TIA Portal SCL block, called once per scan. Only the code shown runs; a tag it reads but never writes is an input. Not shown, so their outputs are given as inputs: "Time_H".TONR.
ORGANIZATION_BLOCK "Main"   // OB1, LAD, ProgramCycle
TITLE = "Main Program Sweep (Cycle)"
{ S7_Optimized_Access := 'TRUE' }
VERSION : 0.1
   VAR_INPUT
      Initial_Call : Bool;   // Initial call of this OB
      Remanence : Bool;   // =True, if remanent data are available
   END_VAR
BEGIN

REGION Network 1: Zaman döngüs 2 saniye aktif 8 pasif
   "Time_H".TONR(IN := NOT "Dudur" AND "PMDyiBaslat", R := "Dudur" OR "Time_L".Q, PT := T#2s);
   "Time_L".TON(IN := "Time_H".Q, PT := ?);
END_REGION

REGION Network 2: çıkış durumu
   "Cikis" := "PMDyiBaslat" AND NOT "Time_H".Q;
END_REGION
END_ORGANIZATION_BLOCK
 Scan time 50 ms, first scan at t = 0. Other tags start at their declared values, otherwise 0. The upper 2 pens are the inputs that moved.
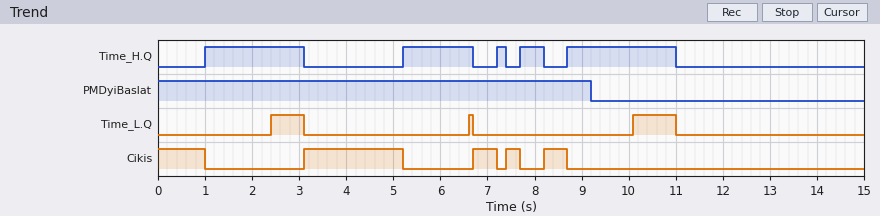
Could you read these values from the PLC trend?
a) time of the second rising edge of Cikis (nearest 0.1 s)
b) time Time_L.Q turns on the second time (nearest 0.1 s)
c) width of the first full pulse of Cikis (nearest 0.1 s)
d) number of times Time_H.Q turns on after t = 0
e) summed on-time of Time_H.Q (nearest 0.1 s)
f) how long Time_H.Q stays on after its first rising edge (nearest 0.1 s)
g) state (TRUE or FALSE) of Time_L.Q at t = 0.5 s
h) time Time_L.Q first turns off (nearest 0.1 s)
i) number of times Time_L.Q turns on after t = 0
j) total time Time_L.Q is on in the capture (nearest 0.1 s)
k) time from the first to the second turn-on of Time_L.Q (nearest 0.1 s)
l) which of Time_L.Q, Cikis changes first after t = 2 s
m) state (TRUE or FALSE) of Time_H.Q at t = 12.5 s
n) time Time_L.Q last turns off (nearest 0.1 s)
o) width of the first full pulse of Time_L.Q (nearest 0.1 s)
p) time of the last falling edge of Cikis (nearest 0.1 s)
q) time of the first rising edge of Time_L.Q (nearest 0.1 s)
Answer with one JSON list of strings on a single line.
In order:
["6.7 s", "6.6 s", "2.1 s", "5", "6.6 s", "2.1 s", "FALSE", "3.1 s", "3", "1.7 s", "4.2 s", "Time_L.Q", "FALSE", "11.0 s", "0.7 s", "8.7 s", "2.4 s"]
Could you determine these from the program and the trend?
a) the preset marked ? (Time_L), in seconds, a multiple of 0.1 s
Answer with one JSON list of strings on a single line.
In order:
["1.4 s"]
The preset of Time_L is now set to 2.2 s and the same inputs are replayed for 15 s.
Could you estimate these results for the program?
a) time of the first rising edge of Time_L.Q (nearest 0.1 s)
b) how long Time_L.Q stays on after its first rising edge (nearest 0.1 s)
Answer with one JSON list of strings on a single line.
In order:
["10.9 s", "0.1 s"]
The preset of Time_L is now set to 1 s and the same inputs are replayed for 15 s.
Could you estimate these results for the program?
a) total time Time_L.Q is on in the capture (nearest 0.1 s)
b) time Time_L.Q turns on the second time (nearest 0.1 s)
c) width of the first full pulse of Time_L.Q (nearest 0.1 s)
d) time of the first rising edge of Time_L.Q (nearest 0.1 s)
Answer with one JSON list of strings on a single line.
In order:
["2.9 s", "6.2 s", "1.1 s", "2.0 s"]
